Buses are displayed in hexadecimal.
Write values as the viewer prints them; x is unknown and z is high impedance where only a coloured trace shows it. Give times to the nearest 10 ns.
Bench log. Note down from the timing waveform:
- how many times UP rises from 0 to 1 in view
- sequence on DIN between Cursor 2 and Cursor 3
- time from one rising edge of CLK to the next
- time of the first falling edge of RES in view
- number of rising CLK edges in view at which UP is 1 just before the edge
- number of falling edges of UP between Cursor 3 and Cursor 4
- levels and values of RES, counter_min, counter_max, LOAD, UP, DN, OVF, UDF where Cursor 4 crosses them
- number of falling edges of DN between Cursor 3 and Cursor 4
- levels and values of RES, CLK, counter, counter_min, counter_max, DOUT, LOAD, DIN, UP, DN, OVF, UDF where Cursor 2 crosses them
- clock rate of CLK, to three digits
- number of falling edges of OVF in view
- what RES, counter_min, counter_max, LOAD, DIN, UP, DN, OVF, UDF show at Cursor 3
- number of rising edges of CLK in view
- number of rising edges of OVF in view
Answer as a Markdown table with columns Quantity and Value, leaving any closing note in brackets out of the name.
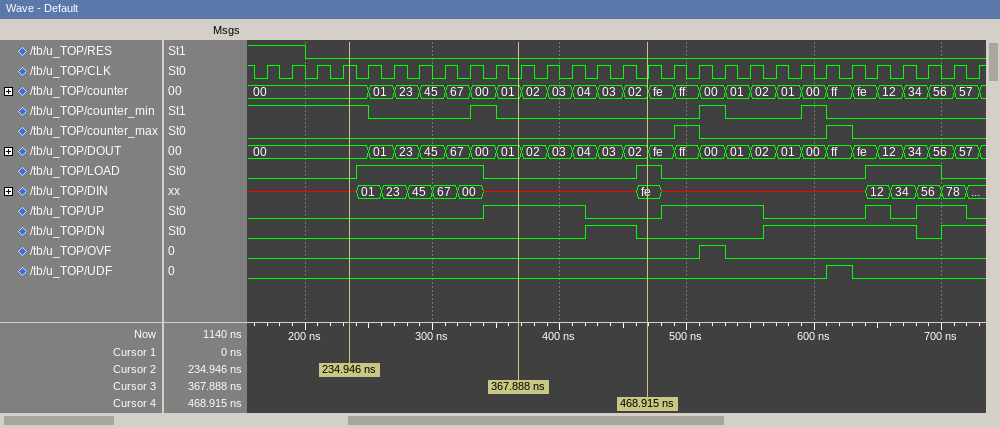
| Quantity | Value |
|---|---|
| how many times UP rises from 0 to 1 in view | 4 |
| sequence on DIN between Cursor 2 and Cursor 3 | x, 01, 23, 45, 67, 00, x |
| time from one rising edge of CLK to the next | 20 ns |
| time of the first falling edge of RES in view | 200 ns |
| number of rising CLK edges in view at which UP is 1 just before the edge | 11 |
| number of falling edges of UP between Cursor 3 and Cursor 4 | 1 |
| levels and values of RES, counter_min, counter_max, LOAD, UP, DN, OVF, UDF where Cursor 4 crosses them | RES=0, counter_min=0, counter_max=0, LOAD=1, UP=0, DN=0, OVF=0, UDF=0 |
| number of falling edges of DN between Cursor 3 and Cursor 4 | 1 |
| levels and values of RES, CLK, counter, counter_min, counter_max, DOUT, LOAD, DIN, UP, DN, OVF, UDF where Cursor 2 crosses them | RES=0, CLK=1, counter=00, counter_min=1, counter_max=0, DOUT=00, LOAD=0, DIN=x, UP=0, DN=0, OVF=0, UDF=0 |
| clock rate of CLK, to three digits | 50.0 MHz |
| number of falling edges of OVF in view | 1 |
| what RES, counter_min, counter_max, LOAD, DIN, UP, DN, OVF, UDF show at Cursor 3 | RES=0, counter_min=0, counter_max=0, LOAD=0, DIN=x, UP=1, DN=0, OVF=0, UDF=0 |
| number of rising edges of CLK in view | 29 |
| number of rising edges of OVF in view | 1 |
